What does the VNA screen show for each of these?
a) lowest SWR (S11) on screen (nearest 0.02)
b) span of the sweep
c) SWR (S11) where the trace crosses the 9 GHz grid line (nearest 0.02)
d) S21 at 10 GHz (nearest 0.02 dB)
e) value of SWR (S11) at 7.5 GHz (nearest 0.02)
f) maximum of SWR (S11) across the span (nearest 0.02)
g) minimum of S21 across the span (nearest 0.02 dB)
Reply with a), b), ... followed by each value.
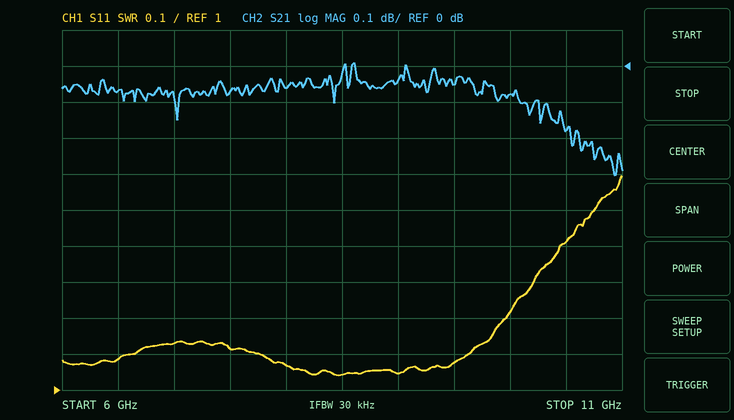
a) 1.04
b) 5 GHz
c) 1.04
d) -0.08 dB
e) 1.12
f) 1.60
g) -0.30 dB
